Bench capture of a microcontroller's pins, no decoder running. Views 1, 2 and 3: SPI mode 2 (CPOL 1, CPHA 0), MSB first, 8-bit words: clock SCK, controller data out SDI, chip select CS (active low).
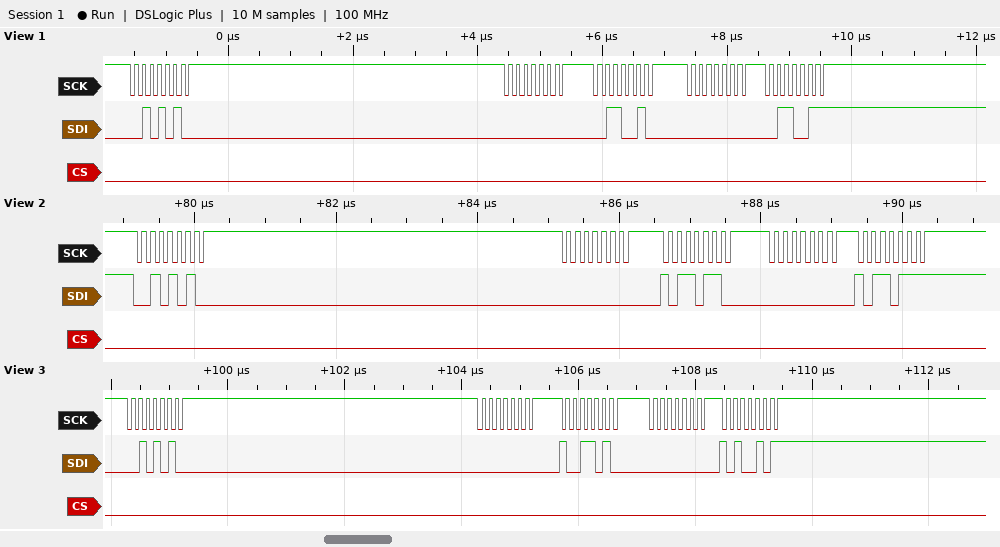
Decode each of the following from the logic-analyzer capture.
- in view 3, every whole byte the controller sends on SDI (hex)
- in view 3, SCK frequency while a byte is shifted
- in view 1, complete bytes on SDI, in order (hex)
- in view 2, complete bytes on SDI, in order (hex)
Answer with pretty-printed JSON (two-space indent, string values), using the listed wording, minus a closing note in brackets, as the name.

{
  "in view 3, every whole byte the controller sends on SDI": "2A 00 9A 00 A5",
  "in view 3, SCK frequency while a byte is shifted": "8 MHz",
  "in view 1, complete bytes on SDI, in order": "2A 00 32 00 33",
  "in view 2, complete bytes on SDI, in order": "2A 00 B6 00 B7"
}
